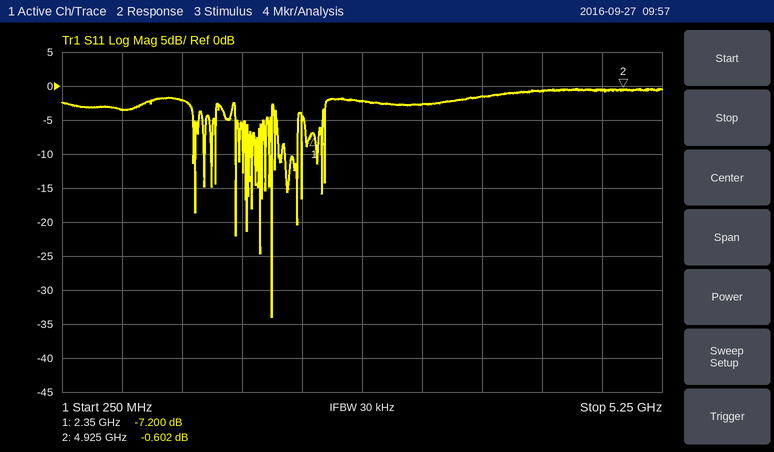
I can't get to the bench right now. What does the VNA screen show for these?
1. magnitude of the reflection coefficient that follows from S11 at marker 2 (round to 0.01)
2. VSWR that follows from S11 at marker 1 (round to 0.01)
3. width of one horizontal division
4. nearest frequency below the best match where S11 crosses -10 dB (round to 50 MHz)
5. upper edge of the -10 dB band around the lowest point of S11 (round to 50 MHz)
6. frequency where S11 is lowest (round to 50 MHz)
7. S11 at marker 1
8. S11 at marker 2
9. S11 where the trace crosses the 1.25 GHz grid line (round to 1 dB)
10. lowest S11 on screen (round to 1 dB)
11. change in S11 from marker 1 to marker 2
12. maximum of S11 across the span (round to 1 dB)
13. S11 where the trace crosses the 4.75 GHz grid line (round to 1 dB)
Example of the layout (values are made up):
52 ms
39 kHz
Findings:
0.93
2.55
500 MHz
2.00 GHz
2.00 GHz
2.00 GHz
-7.200 dB
-0.602 dB
-2 dB
-34 dB
6.598 dB
0 dB
-1 dB
